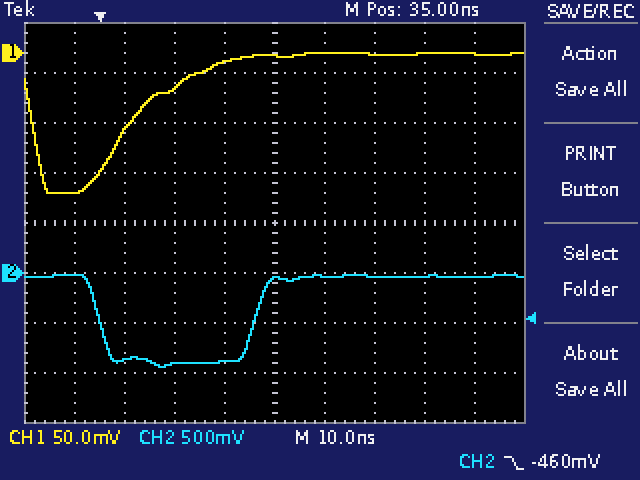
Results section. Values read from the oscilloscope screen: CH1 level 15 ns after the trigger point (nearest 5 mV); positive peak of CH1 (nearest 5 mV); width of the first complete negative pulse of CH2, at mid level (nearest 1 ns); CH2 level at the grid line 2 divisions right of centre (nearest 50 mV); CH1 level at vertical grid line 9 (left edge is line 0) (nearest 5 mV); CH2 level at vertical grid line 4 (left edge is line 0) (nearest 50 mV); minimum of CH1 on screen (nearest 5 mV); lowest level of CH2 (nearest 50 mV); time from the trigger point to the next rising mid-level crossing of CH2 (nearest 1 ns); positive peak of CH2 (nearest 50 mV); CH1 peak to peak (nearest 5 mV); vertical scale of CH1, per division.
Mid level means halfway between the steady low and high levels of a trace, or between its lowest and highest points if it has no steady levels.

-35 mV
0 mV
31 ns
-50 mV
0 mV
-900 mV
-140 mV
-950 mV
31 ns
0 mV
140 mV
50 mV
